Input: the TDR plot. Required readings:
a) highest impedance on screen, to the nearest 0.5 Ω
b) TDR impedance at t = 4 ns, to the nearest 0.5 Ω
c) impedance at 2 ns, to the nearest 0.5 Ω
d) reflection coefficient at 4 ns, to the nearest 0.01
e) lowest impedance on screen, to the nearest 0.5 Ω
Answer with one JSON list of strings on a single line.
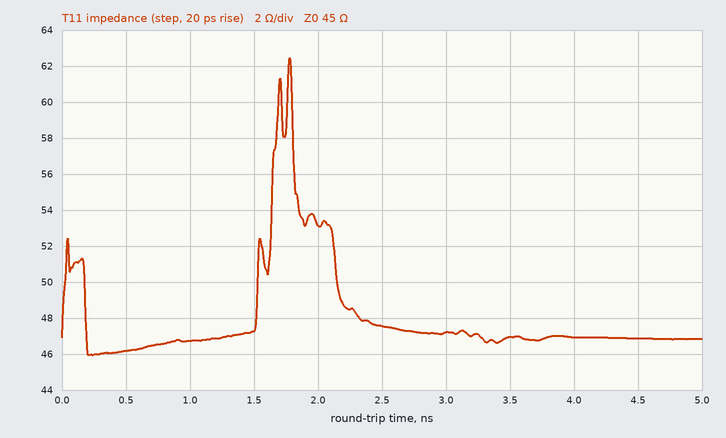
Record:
["62.5 Ω", "47.0 Ω", "53.0 Ω", "+0.02", "46.0 Ω"]
